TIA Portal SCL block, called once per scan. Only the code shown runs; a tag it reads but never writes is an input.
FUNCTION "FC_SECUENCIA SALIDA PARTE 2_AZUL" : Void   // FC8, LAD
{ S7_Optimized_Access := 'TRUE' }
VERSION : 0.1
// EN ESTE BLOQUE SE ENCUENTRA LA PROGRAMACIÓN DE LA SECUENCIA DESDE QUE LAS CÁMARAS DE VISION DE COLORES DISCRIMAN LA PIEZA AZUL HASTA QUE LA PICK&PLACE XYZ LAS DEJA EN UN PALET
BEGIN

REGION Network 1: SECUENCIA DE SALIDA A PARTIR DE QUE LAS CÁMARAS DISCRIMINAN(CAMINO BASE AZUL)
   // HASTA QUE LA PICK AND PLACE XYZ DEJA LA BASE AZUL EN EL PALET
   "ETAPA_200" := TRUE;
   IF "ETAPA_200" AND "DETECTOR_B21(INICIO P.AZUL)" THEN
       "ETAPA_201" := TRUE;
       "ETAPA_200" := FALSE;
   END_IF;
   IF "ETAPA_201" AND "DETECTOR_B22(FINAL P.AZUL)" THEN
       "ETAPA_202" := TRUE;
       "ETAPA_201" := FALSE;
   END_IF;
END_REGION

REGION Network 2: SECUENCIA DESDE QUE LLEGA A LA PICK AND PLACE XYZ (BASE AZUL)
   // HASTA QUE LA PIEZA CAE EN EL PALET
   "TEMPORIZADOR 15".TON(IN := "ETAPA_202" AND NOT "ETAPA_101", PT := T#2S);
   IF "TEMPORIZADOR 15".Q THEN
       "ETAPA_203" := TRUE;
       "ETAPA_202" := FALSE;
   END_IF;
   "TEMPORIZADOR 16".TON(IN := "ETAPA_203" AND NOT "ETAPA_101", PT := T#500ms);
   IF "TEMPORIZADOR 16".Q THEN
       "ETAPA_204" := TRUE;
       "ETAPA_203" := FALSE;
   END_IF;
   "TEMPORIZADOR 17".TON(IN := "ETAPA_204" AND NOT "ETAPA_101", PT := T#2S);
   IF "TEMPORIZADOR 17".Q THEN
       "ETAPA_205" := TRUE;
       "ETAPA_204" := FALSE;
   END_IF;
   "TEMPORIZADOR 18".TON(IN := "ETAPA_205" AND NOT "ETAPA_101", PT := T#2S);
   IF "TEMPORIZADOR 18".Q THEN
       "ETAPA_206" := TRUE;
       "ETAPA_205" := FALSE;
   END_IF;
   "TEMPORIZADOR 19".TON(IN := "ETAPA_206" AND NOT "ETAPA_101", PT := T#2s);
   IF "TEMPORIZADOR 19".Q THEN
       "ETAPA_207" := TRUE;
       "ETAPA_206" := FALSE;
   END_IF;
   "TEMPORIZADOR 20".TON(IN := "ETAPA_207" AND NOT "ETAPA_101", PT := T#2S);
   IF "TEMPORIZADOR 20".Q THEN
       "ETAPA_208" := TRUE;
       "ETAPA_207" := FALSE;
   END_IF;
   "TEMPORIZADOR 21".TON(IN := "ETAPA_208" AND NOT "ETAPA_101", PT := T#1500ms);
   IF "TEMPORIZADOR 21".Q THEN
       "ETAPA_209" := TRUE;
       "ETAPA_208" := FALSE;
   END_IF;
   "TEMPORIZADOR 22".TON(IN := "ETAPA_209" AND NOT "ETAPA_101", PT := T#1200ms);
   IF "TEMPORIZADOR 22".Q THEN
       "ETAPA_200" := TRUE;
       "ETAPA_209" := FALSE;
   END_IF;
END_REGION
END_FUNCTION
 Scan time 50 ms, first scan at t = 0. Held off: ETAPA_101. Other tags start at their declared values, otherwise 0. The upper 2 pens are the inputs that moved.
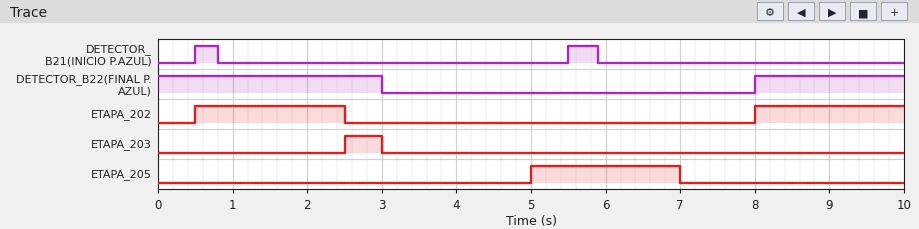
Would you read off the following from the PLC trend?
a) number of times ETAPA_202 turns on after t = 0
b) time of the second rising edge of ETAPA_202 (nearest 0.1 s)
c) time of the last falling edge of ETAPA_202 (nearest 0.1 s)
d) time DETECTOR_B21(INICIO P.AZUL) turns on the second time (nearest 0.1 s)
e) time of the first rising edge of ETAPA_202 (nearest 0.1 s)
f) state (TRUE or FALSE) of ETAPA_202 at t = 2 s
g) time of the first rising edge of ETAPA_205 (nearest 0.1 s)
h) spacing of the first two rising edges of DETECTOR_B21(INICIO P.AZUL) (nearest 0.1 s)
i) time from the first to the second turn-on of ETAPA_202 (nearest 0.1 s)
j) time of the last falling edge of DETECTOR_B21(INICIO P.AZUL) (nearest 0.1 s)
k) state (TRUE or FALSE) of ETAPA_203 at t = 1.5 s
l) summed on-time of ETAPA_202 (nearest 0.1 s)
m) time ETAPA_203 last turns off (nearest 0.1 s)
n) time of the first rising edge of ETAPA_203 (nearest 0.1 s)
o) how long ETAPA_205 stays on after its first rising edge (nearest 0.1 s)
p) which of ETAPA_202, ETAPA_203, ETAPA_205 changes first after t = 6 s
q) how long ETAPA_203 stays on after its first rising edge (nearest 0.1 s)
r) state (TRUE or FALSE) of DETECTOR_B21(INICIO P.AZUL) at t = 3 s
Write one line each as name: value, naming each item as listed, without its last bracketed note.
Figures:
number of times ETAPA_202 turns on after t = 0: 2
time of the second rising edge of ETAPA_202: 8.0 s
time of the last falling edge of ETAPA_202: 2.5 s
time DETECTOR_B21(INICIO P.AZUL) turns on the second time: 5.5 s
time of the first rising edge of ETAPA_202: 0.5 s
state (TRUE or FALSE) of ETAPA_202 at t = 2 s: TRUE
time of the first rising edge of ETAPA_205: 5.0 s
spacing of the first two rising edges of DETECTOR_B21(INICIO P.AZUL): 5.0 s
time from the first to the second turn-on of ETAPA_202: 7.5 s
time of the last falling edge of DETECTOR_B21(INICIO P.AZUL): 5.9 s
state (TRUE or FALSE) of ETAPA_203 at t = 1.5 s: FALSE
summed on-time of ETAPA_202: 4.0 s
time ETAPA_203 last turns off: 3.0 s
time of the first rising edge of ETAPA_203: 2.5 s
how long ETAPA_205 stays on after its first rising edge: 2.0 s
which of ETAPA_202, ETAPA_203, ETAPA_205 changes first after t = 6 s: ETAPA_205
how long ETAPA_203 stays on after its first rising edge: 0.5 s
state (TRUE or FALSE) of DETECTOR_B21(INICIO P.AZUL) at t = 3 s: FALSE
